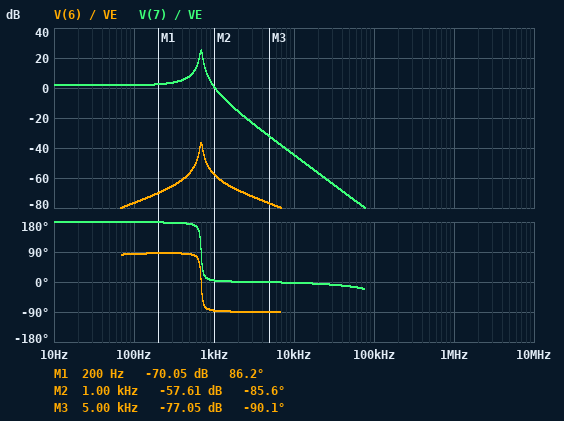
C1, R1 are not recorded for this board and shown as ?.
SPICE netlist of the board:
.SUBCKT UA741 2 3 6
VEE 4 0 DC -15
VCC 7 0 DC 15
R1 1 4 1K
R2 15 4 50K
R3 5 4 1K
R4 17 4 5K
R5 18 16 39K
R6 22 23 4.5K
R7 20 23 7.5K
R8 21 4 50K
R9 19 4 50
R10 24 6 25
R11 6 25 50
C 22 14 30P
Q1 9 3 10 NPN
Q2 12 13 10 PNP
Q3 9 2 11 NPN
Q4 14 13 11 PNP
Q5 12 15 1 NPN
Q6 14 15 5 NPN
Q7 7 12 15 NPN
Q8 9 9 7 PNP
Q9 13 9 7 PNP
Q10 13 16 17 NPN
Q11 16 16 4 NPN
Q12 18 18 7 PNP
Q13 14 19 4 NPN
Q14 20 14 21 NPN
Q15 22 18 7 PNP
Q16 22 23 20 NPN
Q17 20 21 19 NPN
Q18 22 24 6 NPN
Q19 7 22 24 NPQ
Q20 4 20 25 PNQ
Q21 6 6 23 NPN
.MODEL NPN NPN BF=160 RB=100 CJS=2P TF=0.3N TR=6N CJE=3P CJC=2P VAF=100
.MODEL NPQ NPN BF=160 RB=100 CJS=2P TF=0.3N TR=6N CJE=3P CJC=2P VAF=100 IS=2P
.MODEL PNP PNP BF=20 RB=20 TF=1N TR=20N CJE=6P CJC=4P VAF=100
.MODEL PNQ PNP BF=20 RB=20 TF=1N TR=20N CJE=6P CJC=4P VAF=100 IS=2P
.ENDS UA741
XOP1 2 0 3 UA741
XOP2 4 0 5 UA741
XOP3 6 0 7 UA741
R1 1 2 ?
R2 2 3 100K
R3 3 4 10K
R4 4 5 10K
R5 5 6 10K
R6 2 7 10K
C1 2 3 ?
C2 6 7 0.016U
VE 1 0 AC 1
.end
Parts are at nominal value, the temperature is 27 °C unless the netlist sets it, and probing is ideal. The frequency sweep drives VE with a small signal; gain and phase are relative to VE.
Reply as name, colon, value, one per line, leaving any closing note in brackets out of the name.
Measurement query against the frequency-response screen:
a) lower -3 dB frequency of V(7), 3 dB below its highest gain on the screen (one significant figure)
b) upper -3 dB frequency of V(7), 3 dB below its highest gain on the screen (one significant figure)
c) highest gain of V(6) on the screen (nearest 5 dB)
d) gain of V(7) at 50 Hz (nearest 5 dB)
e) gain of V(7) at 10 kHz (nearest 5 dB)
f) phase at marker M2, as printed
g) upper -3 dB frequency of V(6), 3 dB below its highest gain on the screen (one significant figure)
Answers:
lower -3 dB frequency of V(7), 3 dB below its highest gain on the screen: 700 Hz
upper -3 dB frequency of V(7), 3 dB below its highest gain on the screen: 700 Hz
highest gain of V(6) on the screen: -35 dB
gain of V(7) at 50 Hz: 0 dB
gain of V(7) at 10 kHz: -45 dB
phase at marker M2, as printed: -85.6 deg
upper -3 dB frequency of V(6), 3 dB below its highest gain on the screen: 700 Hz
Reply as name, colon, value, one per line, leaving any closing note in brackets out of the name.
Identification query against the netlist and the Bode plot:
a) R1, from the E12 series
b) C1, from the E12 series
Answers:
R1, from the E12 series: 8.2 kΩ
C1, from the E12 series: 33 nF
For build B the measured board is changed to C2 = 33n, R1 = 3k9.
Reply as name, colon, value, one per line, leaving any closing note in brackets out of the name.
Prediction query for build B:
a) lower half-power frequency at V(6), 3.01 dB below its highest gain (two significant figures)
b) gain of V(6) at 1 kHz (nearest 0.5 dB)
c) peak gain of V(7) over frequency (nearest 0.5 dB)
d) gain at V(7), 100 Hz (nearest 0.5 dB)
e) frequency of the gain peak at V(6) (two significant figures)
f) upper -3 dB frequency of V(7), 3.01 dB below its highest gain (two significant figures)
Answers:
lower half-power frequency at V(6), 3.01 dB below its highest gain: 460 Hz
gain of V(6) at 1 kHz: -61.0 dB
peak gain of V(7) over frequency: 28.5 dB
gain at V(7), 100 Hz: 8.5 dB
frequency of the gain peak at V(6): 480 Hz
upper -3 dB frequency of V(7), 3.01 dB below its highest gain: 500 Hz
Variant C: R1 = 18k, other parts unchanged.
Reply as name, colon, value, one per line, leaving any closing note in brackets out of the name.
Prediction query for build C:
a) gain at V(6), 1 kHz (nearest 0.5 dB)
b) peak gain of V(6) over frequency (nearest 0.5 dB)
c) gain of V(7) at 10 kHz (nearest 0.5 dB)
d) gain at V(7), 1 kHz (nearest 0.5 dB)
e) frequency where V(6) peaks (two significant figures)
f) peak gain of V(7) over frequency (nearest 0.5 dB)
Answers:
gain at V(6), 1 kHz: -64.5 dB
peak gain of V(6) over frequency: -43.5 dB
gain of V(7) at 10 kHz: -51.5 dB
gain at V(7), 1 kHz: -6.0 dB
frequency where V(6) peaks: 690 Hz
peak gain of V(7) over frequency: 18.5 dB
